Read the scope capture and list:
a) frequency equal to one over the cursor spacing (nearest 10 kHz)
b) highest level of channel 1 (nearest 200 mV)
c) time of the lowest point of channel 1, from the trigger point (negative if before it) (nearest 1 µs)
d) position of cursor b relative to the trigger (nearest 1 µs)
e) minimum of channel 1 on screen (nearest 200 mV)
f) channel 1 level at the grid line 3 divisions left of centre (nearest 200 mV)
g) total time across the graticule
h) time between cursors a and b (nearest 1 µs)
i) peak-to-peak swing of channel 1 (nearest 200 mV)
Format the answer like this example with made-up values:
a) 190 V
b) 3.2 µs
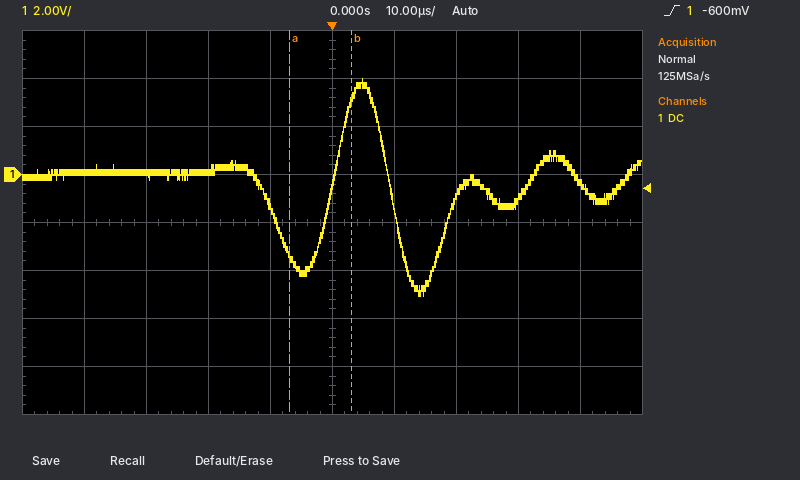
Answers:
a) 100 kHz
b) 4.0 V
c) +14 µs
d) +3 µs
e) -5.0 V
f) 0.0 V
g) 100 µs
h) 10 µs
i) 9.0 V
